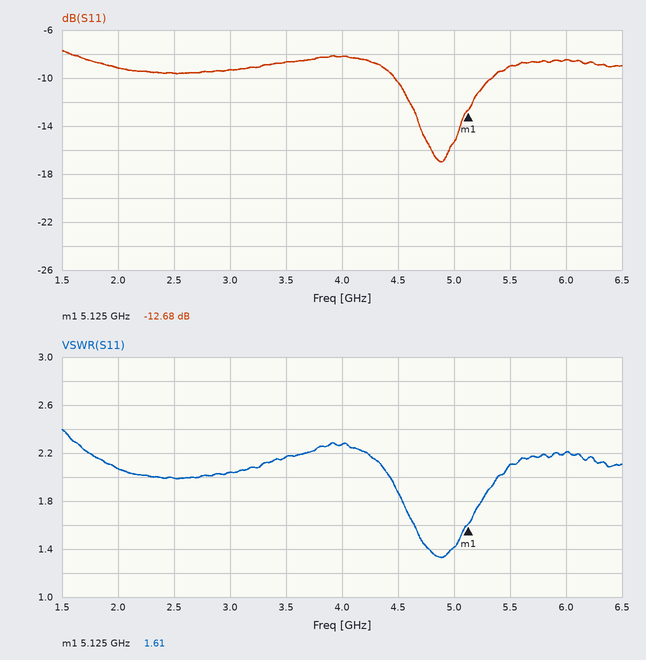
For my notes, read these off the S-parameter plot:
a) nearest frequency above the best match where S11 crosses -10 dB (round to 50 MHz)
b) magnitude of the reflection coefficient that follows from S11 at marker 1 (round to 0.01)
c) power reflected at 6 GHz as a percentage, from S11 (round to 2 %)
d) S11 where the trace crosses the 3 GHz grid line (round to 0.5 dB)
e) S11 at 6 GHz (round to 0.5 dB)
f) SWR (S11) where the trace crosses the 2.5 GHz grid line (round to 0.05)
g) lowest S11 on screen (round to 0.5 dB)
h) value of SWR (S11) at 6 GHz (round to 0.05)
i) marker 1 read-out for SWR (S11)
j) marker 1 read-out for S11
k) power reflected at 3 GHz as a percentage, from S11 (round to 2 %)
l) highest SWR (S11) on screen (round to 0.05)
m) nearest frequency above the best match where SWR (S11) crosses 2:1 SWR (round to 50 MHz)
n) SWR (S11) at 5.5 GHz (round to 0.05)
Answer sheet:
5.35 GHz
0.23
14 %
-9.5 dB
-8.5 dB
2.00
-17.0 dB
2.20
1.61
-12.68 dB
12 %
2.40
5.40 GHz
2.10
